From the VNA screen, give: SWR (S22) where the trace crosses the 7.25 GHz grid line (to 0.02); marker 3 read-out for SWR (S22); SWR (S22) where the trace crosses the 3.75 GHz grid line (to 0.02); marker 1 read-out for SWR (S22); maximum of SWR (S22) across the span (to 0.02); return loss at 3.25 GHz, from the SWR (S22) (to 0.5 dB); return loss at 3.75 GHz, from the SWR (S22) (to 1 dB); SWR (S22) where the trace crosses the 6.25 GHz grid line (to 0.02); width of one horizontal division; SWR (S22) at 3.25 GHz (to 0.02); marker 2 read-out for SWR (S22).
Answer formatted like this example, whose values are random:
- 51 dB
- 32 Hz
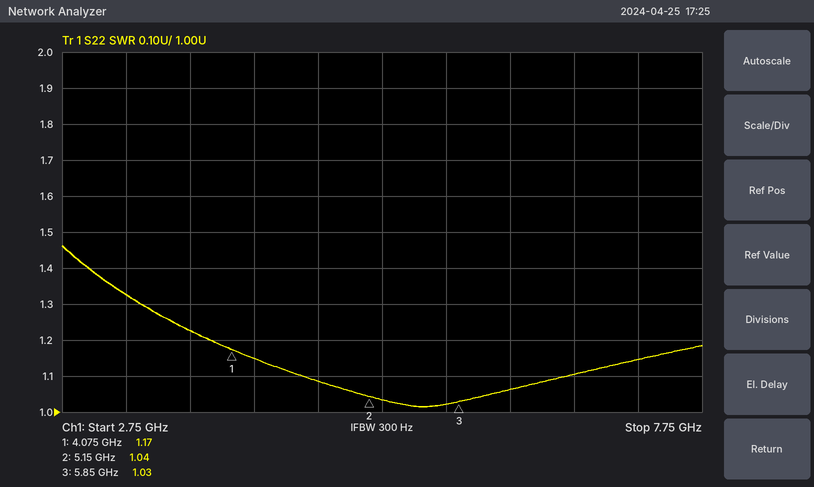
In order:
- 1.14
- 1.03
- 1.22
- 1.17
- 1.46
- 17.0 dB
- 20 dB
- 1.06
- 500 MHz
- 1.32
- 1.04
